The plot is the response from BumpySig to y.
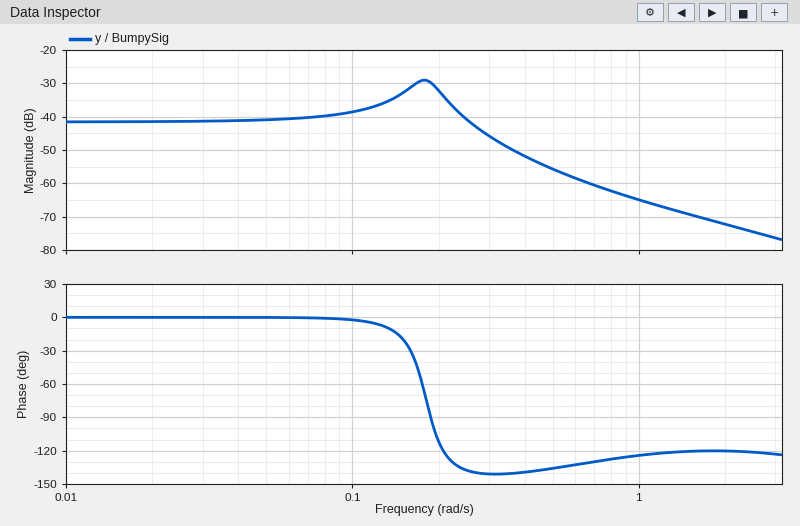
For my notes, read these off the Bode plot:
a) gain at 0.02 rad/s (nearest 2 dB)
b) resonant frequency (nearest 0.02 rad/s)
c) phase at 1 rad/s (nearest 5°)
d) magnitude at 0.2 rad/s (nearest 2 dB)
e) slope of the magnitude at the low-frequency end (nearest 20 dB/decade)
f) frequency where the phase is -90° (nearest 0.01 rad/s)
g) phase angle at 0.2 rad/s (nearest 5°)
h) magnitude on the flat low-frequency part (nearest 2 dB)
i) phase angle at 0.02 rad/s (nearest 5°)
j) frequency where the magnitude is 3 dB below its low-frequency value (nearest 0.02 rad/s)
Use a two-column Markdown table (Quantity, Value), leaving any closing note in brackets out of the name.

| Quantity | Value |
|---|---|
| gain at 0.02 rad/s | -42 dB |
| resonant frequency | 0.18 rad/s |
| phase at 1 rad/s | -125° |
| magnitude at 0.2 rad/s | -32 dB |
| slope of the magnitude at the low-frequency end | 0 dB/decade |
| frequency where the phase is -90° | 0.19 rad/s |
| phase angle at 0.2 rad/s | -110° |
| magnitude on the flat low-frequency part | -42 dB |
| phase angle at 0.02 rad/s | 0° |
| frequency where the magnitude is 3 dB below its low-frequency value | 0.28 rad/s |
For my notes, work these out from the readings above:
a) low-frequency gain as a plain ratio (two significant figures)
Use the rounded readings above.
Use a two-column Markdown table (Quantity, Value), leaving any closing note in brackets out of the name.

| Quantity | Value |
|---|---|
| low-frequency gain as a plain ratio | 0.0079 |
